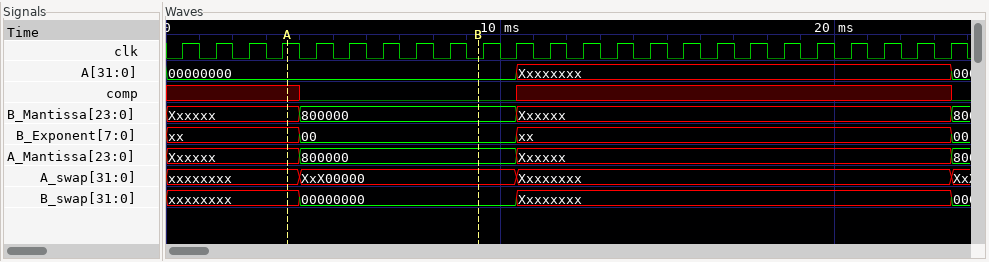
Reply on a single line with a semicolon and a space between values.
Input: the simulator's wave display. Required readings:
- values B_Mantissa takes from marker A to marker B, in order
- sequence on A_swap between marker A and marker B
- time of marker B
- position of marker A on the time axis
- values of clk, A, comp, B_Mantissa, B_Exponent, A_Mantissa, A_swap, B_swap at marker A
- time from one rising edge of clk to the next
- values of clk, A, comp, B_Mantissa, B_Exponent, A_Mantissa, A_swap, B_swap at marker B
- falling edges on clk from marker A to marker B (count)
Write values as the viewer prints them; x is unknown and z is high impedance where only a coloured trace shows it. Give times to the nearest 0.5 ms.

Xxxxxx, 800000; xxxxxxxx, XxX00000; 9.5 ms; 3.5 ms; clk=1, A=00000000, comp=x, B_Mantissa=Xxxxxx, B_Exponent=xx, A_Mantissa=Xxxxxx, A_swap=xxxxxxxx, B_swap=xxxxxxxx; 1 ms; clk=0, A=00000000, comp=0, B_Mantissa=800000, B_Exponent=00, A_Mantissa=800000, A_swap=XxX00000, B_swap=00000000; 6
